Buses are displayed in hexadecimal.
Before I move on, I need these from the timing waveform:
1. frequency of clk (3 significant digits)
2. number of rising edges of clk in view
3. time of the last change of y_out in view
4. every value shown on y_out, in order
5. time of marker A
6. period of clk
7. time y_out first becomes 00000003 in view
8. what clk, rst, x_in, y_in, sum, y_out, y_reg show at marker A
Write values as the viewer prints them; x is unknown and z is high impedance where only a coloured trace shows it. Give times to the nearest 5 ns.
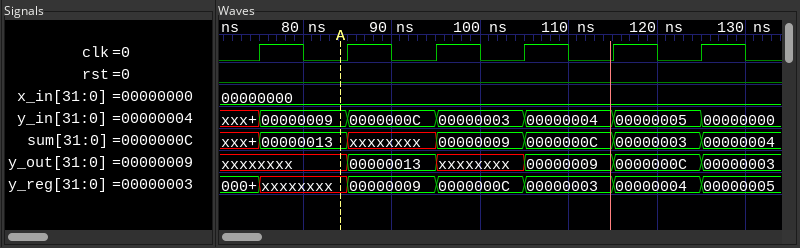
100 MHz
6
125 ns
xxxxxxxx, 00000013, xxxxxxxx, 00000009, 0000000C, 00000003
85 ns
10 ns
125 ns
clk=0, rst=0, x_in=00000000, y_in=00000009, sum=00000013, y_out=xxxxxxxx, y_reg=xxxxxxxx
